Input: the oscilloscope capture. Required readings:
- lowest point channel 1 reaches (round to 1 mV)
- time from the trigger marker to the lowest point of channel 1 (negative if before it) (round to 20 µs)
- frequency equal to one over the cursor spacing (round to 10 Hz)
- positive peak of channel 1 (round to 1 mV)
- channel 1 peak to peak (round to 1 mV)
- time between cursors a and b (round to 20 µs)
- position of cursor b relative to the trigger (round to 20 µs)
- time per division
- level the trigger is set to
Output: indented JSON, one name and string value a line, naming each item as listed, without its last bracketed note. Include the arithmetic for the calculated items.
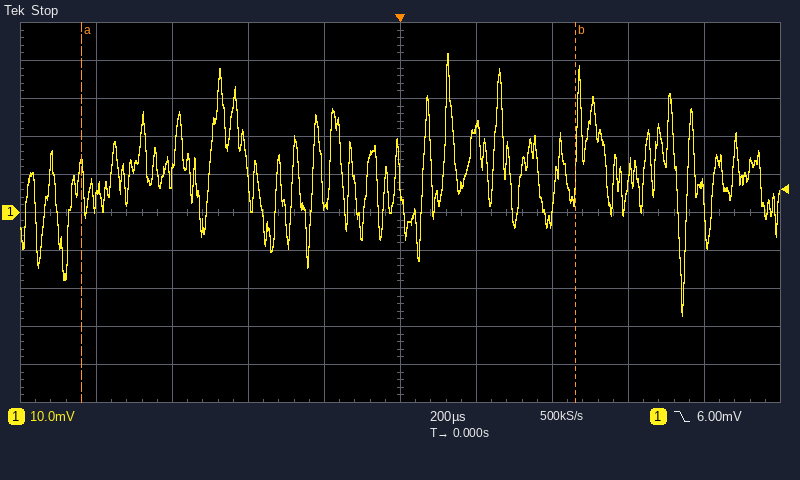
{
  "lowest point channel 1 reaches": "-27 mV",
  "time from the trigger marker to the lowest point of channel 1 (negative if before it)": "+740 µs",
  "frequency equal to one over the cursor spacing": "1 / 1.30 ms ≈ 770 Hz",
  "positive peak of channel 1": "42 mV",
  "channel 1 peak to peak": "42 mV − (-27 mV) = 69 mV",
  "time between cursors a and b": "1.30 ms",
  "position of cursor b relative to the trigger": "+460 µs",
  "time per division": "200 µs",
  "level the trigger is set to": "6.00 mV"
}
